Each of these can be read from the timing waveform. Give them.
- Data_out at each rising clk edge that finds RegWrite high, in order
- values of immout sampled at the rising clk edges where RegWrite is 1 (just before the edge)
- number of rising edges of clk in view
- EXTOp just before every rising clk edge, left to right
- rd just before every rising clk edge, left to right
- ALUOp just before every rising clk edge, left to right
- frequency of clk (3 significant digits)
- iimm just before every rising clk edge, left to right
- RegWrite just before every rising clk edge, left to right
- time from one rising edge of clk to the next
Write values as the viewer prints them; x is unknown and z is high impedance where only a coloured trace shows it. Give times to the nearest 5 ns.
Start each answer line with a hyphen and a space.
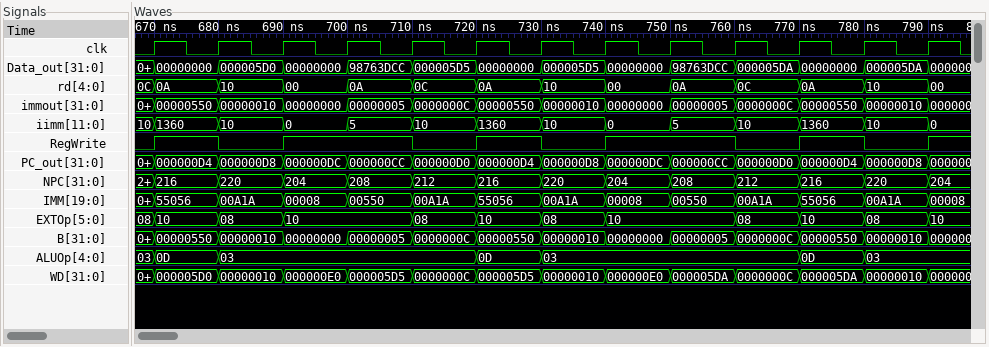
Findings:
- 00000000, 00000000, 98763DCC, 00000000, 00000000, 98763DCC, 00000000
- 00000550, 00000000, 00000005, 00000550, 00000000, 00000005, 00000550
- 13
- 08, 10, 08, 10, 10, 08, 10, 08, 10, 10, 08, 10, 08
- 0C, 0A, 10, 00, 0A, 0C, 0A, 10, 00, 0A, 0C, 0A, 10
- 03, 0D, 03, 03, 03, 03, 0D, 03, 03, 03, 03, 0D, 03
- 100 MHz
- 10, 1360, 10, 0, 5, 10, 1360, 10, 0, 5, 10, 1360, 10
- 0 1 0 1 1 0 1 0 1 1 0 1 0
- 10 ns
